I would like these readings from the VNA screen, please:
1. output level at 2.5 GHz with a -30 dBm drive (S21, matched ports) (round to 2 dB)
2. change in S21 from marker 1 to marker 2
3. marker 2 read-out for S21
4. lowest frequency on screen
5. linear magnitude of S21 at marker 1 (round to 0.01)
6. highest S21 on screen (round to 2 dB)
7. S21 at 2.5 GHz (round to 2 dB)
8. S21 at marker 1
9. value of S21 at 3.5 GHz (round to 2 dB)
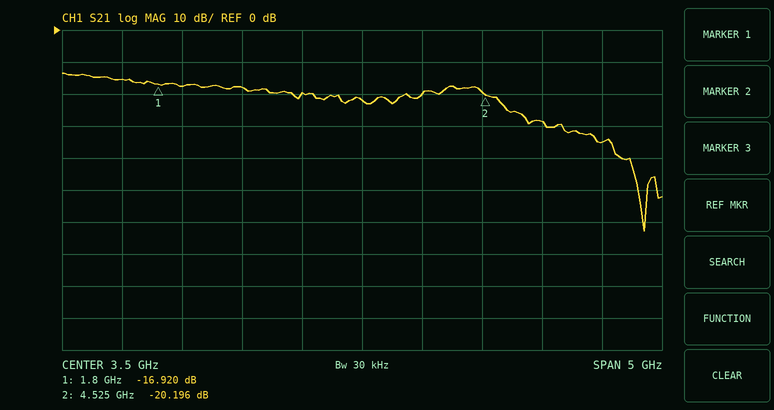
-48 dBm
-3.276 dB
-20.196 dB
1 GHz
0.14
-14 dB
-18 dB
-16.920 dB
-22 dB
